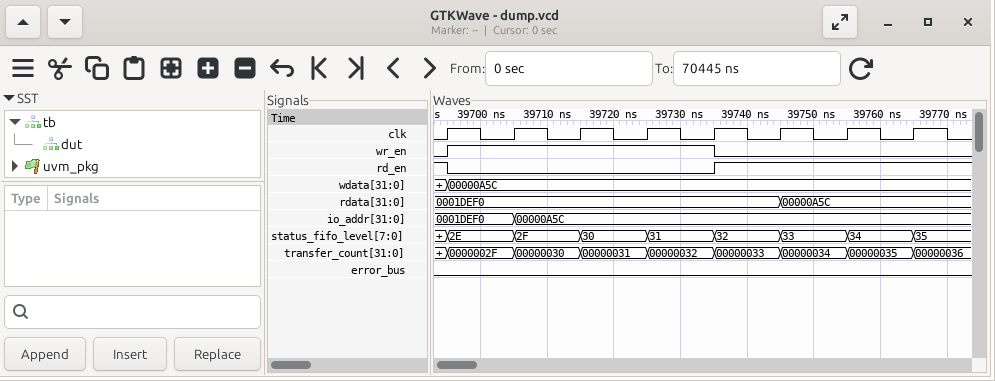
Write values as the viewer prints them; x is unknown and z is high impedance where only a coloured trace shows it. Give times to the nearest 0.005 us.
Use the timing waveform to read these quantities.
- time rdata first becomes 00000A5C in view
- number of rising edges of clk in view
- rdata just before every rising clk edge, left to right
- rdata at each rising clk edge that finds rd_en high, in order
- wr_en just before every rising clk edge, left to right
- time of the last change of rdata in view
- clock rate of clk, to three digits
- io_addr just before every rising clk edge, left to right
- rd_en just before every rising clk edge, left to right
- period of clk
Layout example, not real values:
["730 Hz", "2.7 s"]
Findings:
["39.745 us", "8", "0001DEF0, 0001DEF0, 0001DEF0, 0001DEF0, 0001DEF0, 0001DEF0, 00000A5C, 00000A5C", "0001DEF0, 0001DEF0, 00000A5C, 00000A5C", "0 1 1 1 1 0 0 0", "39.745 us", "100 MHz", "0001DEF0, 0001DEF0, 00000A5C, 00000A5C, 00000A5C, 00000A5C, 00000A5C, 00000A5C", "1 0 0 0 0 1 1 1", "0.01 us"]
